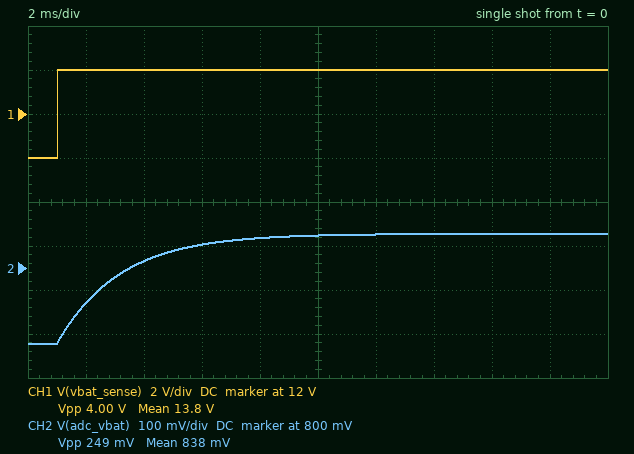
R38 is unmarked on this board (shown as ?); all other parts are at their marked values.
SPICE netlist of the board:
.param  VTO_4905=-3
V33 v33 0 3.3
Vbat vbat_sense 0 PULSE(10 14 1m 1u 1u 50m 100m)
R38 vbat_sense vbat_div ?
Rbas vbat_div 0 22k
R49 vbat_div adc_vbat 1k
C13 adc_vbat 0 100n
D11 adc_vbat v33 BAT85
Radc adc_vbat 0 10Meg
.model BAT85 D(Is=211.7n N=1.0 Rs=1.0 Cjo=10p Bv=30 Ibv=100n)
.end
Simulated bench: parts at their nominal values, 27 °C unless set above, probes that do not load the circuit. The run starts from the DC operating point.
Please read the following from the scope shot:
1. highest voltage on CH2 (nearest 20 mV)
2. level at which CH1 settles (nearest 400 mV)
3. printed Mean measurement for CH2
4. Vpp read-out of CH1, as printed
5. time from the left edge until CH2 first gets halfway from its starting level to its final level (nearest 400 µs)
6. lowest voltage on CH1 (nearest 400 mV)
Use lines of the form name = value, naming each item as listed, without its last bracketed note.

highest voltage on CH2 = 880 mV
level at which CH1 settles = 14.0 V
printed Mean measurement for CH2 = 838 mV
Vpp read-out of CH1, as printed = 4.00 V
time from the left edge until CH2 first gets halfway from its starting level to its final level = 2.4 ms
lowest voltage on CH1 = 10.0 V
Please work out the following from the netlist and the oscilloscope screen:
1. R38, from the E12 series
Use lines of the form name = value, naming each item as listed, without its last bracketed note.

R38, from the E12 series = 330 kΩ
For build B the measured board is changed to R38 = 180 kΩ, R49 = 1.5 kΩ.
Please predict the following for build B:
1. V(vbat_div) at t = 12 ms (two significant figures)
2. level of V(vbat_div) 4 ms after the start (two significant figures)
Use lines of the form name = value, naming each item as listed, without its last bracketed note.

V(vbat_div) at t = 12 ms = 1.5 V
level of V(vbat_div) 4 ms after the start = 1.4 V
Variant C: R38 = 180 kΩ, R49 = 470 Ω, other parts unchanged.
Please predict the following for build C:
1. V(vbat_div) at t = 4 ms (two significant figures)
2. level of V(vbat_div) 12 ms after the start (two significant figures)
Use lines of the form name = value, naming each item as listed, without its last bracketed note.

V(vbat_div) at t = 4 ms = 1.4 V
level of V(vbat_div) 12 ms after the start = 1.5 V
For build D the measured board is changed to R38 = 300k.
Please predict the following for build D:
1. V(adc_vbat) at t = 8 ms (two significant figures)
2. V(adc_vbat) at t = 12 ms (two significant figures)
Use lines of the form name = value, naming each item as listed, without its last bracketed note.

V(adc_vbat) at t = 8 ms = 950 mV
V(adc_vbat) at t = 12 ms = 960 mV
